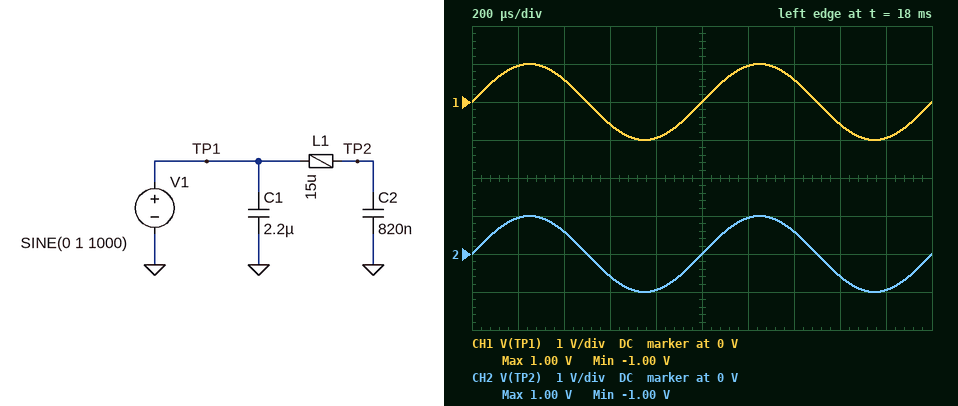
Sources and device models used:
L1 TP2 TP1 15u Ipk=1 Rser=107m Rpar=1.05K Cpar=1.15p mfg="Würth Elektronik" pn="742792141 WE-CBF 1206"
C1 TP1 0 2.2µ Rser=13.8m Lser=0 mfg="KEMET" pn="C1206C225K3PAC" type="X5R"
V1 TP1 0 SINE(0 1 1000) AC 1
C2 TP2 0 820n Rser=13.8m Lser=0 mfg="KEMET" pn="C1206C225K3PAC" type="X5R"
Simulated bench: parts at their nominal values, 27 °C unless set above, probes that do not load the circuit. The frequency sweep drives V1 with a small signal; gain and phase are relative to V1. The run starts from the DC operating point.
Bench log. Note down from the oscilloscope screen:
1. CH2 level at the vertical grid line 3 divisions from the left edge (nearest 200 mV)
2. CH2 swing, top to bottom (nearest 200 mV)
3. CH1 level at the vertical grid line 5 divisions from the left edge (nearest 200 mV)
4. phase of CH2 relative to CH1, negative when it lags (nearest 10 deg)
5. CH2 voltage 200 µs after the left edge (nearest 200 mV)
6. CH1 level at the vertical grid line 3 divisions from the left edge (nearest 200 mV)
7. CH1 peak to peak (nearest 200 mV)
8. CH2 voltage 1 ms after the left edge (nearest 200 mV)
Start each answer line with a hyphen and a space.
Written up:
- -600 mV
- 2.0 V
- 0 V
- 0 deg
- 1.0 V
- -600 mV
- 2.0 V
- 0 V
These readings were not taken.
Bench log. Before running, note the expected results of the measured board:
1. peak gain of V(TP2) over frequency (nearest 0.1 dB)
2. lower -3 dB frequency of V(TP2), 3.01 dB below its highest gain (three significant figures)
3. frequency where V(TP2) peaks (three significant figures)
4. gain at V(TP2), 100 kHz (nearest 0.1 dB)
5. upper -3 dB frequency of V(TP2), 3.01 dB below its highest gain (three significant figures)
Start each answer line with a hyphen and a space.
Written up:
- 29.8 dB
- 44.6 kHz
- 45.4 kHz
- -11.7 dB
- 46.1 kHz
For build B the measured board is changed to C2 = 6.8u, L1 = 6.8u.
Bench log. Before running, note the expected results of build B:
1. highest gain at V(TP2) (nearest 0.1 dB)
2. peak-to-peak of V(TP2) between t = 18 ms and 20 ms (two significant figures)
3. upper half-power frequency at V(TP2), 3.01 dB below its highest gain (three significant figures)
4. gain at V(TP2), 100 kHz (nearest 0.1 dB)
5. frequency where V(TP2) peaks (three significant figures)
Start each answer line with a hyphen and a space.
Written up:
- 18.3 dB
- 2.0 V
- 24.7 kHz
- -24.7 dB
- 23.3 kHz
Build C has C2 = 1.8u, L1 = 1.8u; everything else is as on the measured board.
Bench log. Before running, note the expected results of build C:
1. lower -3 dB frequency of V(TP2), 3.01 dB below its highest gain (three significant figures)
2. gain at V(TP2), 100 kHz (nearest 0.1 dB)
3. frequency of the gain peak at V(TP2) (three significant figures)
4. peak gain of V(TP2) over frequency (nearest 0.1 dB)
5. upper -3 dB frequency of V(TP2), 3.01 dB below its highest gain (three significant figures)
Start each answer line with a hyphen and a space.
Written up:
- 82.5 kHz
- 10.1 dB
- 88.1 kHz
- 18.3 dB
- 93.3 kHz
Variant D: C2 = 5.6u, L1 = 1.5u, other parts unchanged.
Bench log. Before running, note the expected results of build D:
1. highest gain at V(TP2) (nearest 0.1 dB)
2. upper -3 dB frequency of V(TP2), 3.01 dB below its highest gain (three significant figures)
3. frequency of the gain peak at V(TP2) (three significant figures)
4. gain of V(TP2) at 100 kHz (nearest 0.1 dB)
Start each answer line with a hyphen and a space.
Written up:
- 12.7 dB
- 60.3 kHz
- 54.2 kHz
- -7.4 dB
